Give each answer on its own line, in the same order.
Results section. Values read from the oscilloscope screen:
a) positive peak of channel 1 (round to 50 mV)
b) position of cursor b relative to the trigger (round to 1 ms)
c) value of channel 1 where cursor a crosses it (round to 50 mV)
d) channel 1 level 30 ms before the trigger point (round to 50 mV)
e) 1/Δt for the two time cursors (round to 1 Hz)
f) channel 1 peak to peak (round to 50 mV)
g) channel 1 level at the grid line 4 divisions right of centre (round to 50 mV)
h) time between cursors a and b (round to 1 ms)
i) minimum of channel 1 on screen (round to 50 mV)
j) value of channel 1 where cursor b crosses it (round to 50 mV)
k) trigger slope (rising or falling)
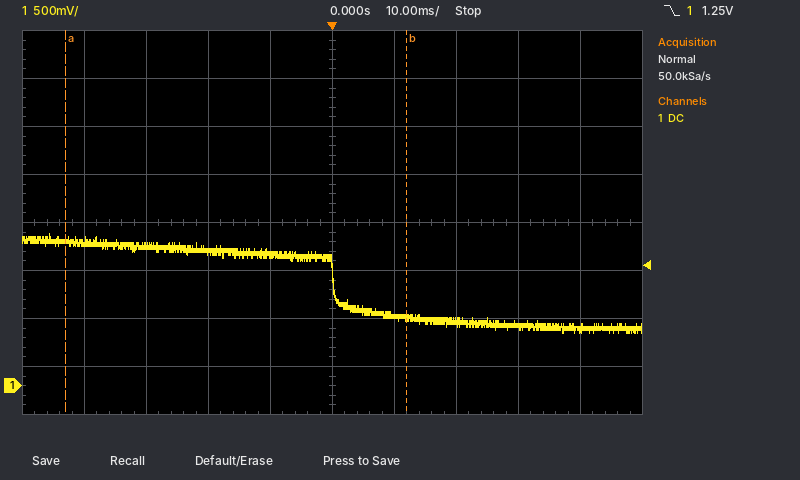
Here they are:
1.60 V
+12 ms
1.50 V
1.45 V
18 Hz
1.05 V
600 mV
55 ms
550 mV
700 mV
falling
